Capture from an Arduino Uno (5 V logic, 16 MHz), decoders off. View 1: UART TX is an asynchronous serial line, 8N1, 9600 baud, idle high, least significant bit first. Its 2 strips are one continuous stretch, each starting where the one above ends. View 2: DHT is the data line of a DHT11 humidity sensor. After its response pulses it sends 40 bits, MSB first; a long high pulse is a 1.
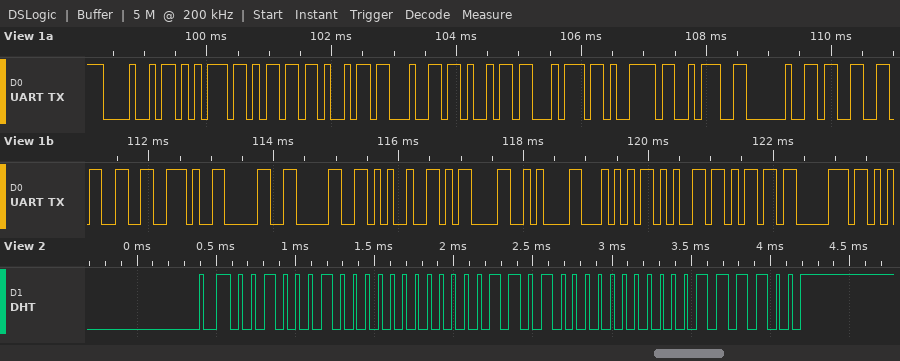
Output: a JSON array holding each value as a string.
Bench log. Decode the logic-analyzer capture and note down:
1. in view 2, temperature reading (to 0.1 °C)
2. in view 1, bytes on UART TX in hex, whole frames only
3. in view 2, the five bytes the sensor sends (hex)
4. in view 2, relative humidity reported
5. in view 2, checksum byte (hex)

["26.0 °C", "48 75 6D 69 64 69 74 79 3A 20 33 33 2E 30 30 25 0D 0A 54 65 6D 70", "22 00 1A 00 3C", "34 %", "0x3C"]
